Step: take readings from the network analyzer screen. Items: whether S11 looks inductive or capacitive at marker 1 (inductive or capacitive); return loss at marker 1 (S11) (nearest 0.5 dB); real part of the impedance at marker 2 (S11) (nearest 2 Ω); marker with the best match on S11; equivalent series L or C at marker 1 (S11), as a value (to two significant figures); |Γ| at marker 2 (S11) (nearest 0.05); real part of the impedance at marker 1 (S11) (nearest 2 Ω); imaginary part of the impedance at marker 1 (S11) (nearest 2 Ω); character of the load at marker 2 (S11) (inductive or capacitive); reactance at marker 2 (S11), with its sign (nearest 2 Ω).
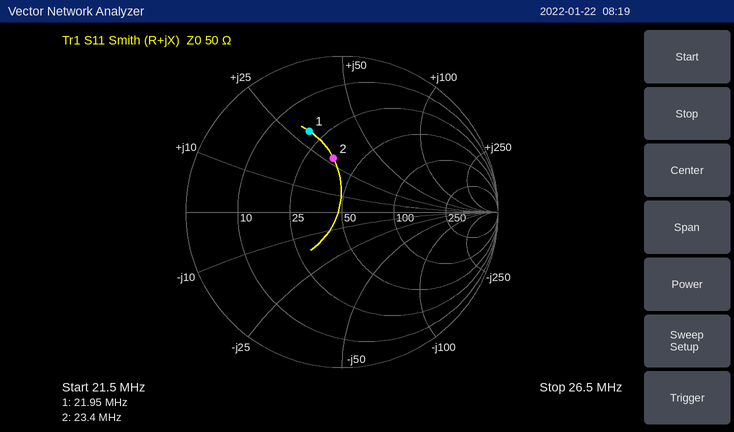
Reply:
inductive
5.0 dB
36 Ω
marker 2
220 nH
0.35
20 Ω
+30 Ω
inductive
+28 Ω
